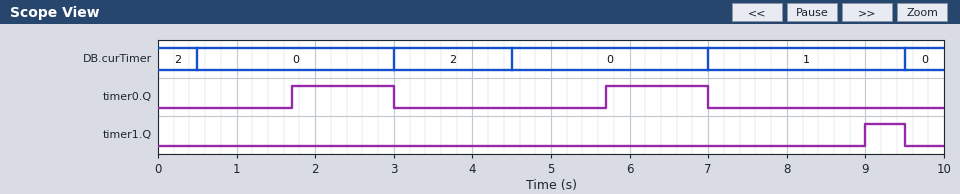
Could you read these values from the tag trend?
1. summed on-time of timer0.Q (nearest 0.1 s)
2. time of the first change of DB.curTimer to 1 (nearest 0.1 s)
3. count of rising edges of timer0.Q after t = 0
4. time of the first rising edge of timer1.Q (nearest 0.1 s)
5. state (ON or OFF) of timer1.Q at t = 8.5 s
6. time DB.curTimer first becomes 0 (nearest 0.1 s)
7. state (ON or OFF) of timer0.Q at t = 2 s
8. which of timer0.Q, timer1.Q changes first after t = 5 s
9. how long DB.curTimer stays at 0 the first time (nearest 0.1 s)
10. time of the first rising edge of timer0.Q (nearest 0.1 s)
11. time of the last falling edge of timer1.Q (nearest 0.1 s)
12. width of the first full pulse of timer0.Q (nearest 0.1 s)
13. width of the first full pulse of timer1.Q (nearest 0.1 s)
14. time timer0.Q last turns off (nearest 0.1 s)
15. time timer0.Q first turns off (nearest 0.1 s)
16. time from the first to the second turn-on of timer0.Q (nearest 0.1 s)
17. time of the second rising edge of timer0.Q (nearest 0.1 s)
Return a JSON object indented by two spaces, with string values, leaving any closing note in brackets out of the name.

{
  "summed on-time of timer0.Q": "2.6 s",
  "time of the first change of DB.curTimer to 1": "7.0 s",
  "count of rising edges of timer0.Q after t = 0": "2",
  "time of the first rising edge of timer1.Q": "9.0 s",
  "state (ON or OFF) of timer1.Q at t = 8.5 s": "OFF",
  "time DB.curTimer first becomes 0": "0.5 s",
  "state (ON or OFF) of timer0.Q at t = 2 s": "ON",
  "which of timer0.Q, timer1.Q changes first after t = 5 s": "timer0.Q",
  "how long DB.curTimer stays at 0 the first time": "2.5 s",
  "time of the first rising edge of timer0.Q": "1.7 s",
  "time of the last falling edge of timer1.Q": "9.5 s",
  "width of the first full pulse of timer0.Q": "1.3 s",
  "width of the first full pulse of timer1.Q": "0.5 s",
  "time timer0.Q last turns off": "7.0 s",
  "time timer0.Q first turns off": "3.0 s",
  "time from the first to the second turn-on of timer0.Q": "4.0 s",
  "time of the second rising edge of timer0.Q": "5.7 s"
}
